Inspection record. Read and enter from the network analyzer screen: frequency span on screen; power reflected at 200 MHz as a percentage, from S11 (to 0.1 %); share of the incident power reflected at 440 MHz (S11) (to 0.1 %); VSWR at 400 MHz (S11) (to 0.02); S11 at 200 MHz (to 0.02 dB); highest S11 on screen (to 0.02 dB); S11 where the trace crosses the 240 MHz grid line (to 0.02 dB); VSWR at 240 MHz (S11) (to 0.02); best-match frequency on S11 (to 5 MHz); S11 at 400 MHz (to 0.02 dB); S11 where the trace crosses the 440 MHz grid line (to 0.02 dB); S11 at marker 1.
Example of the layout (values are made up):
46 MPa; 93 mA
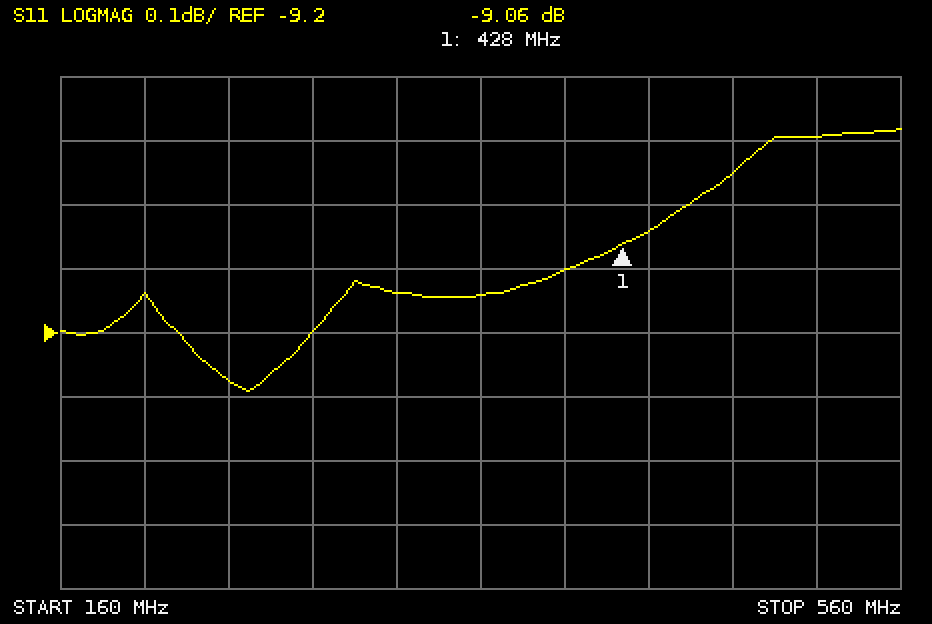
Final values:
400 MHz; 12.2 %; 12.5 %; 2.08; -9.14 dB; -8.88 dB; -9.28 dB; 2.04; 250 MHz; -9.10 dB; -9.04 dB; -9.06 dB
